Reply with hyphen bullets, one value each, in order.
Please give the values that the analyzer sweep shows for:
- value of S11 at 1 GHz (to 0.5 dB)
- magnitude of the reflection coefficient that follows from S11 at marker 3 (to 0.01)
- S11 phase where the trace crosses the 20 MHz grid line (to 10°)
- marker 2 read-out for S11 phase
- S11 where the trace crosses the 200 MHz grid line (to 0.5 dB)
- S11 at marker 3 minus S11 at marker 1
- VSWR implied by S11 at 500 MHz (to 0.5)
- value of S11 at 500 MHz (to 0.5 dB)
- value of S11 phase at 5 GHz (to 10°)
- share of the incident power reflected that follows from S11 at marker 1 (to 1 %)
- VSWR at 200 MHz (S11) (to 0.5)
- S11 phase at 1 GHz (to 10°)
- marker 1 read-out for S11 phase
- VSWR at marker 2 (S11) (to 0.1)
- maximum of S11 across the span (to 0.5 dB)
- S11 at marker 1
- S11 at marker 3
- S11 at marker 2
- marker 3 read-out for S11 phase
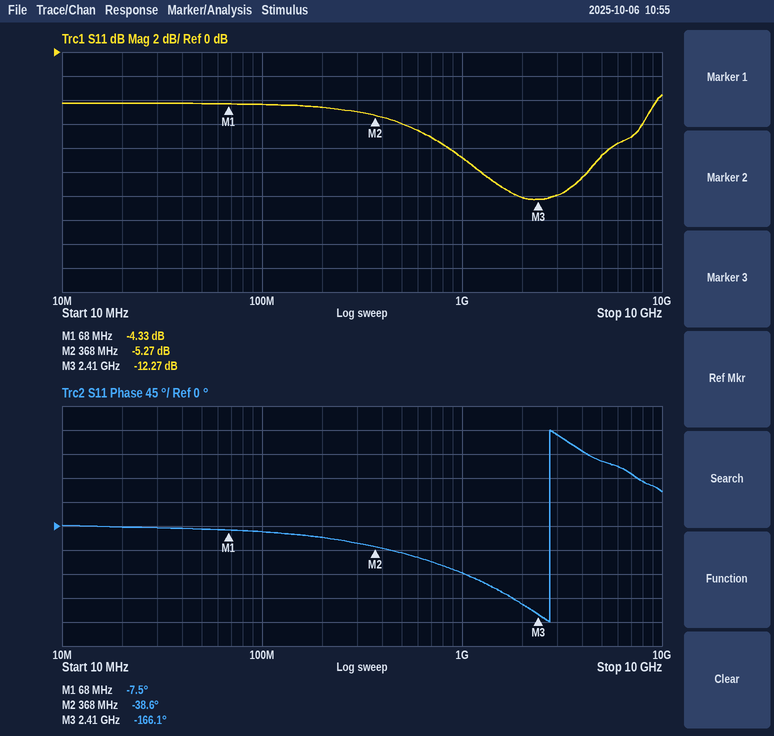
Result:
- -9.0 dB
- 0.24
- 0°
- -38.6°
- -4.5 dB
- -7.94 dB
- 3.0
- -6.0 dB
- 120°
- 37 %
- 4.0
- -90°
- -7.5°
- 3.4
- -3.5 dB
- -4.33 dB
- -12.27 dB
- -5.27 dB
- -166.1°
